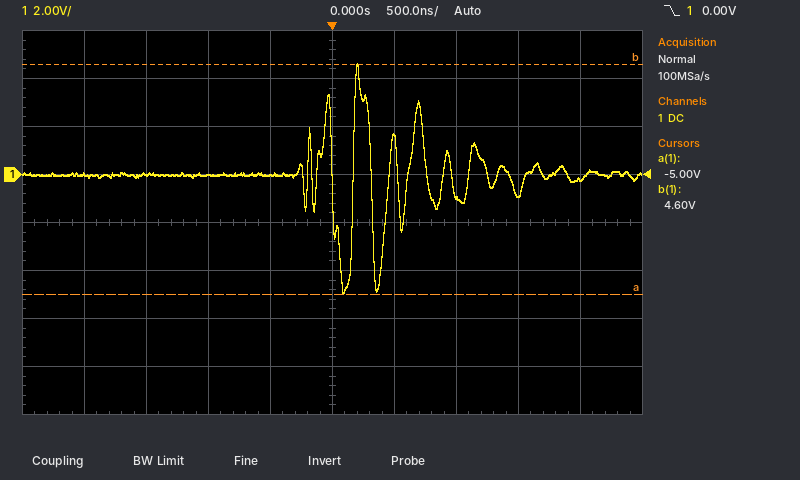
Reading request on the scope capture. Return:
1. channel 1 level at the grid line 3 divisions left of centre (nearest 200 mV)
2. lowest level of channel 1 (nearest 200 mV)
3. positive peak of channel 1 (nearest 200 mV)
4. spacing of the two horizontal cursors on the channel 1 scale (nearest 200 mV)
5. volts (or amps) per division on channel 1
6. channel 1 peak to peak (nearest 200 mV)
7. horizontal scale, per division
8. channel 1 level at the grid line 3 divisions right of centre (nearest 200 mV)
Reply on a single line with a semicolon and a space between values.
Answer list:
0.0 V; -5.0 V; 4.6 V; 9.6 V; 2 V; 9.6 V; 500 ns; -800 mV
